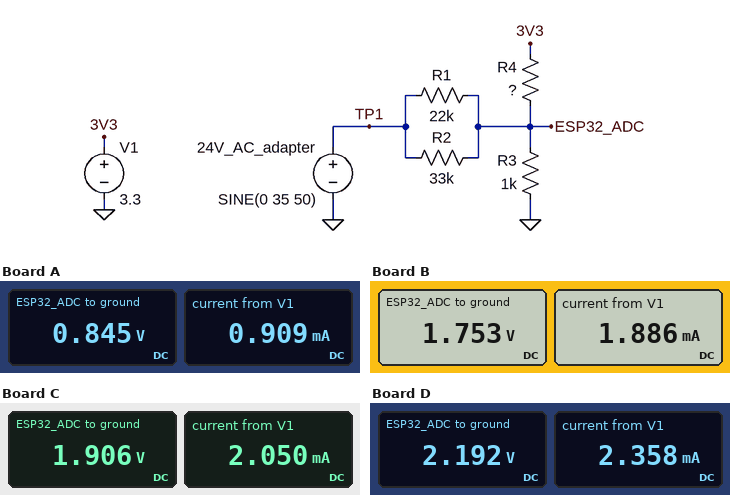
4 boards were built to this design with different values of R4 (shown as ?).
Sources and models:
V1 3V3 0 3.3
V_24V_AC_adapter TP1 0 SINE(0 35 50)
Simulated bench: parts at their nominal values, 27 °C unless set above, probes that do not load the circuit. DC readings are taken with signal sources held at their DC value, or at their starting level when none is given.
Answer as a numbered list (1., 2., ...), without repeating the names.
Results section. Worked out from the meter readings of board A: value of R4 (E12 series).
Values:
1. 2.7 kΩ
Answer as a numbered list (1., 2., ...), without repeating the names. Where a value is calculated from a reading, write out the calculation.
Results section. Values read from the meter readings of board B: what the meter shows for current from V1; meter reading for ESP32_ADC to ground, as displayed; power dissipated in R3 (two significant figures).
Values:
1. 1.886 mA
2. 1.753 V
3. (1.753 V)^2 / 1 kΩ = 3.1 mW
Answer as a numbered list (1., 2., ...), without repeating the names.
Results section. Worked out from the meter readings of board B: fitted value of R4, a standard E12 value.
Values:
1. 820 Ω
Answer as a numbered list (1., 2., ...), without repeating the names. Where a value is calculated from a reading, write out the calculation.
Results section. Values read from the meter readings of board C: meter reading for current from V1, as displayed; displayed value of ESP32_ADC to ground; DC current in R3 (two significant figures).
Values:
1. 2.050 mA
2. 1.906 V
3. (1.906 V) / 1 kΩ = 1.9 mA
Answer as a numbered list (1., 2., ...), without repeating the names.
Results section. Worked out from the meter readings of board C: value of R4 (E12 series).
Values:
1. 680 Ω
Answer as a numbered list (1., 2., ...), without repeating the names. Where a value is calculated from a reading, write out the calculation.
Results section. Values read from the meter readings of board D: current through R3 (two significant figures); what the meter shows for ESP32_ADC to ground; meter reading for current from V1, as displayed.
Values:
1. (2.192 V) / 1 kΩ = 2.2 mA
2. 2.192 V
3. 2.358 mA
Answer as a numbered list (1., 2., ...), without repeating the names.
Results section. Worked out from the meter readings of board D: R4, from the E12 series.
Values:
1. 470 Ω
